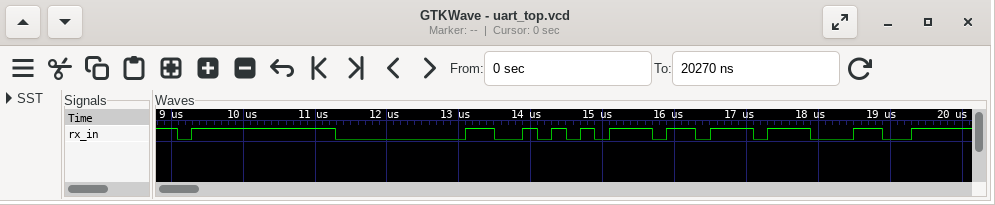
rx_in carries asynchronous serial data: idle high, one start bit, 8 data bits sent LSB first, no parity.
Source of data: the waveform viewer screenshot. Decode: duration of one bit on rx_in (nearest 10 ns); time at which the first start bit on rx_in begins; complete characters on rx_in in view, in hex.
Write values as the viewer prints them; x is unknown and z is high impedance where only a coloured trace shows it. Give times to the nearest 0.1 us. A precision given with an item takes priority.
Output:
200 ns
9.1 us
FF, 00, AA, BB, CC
